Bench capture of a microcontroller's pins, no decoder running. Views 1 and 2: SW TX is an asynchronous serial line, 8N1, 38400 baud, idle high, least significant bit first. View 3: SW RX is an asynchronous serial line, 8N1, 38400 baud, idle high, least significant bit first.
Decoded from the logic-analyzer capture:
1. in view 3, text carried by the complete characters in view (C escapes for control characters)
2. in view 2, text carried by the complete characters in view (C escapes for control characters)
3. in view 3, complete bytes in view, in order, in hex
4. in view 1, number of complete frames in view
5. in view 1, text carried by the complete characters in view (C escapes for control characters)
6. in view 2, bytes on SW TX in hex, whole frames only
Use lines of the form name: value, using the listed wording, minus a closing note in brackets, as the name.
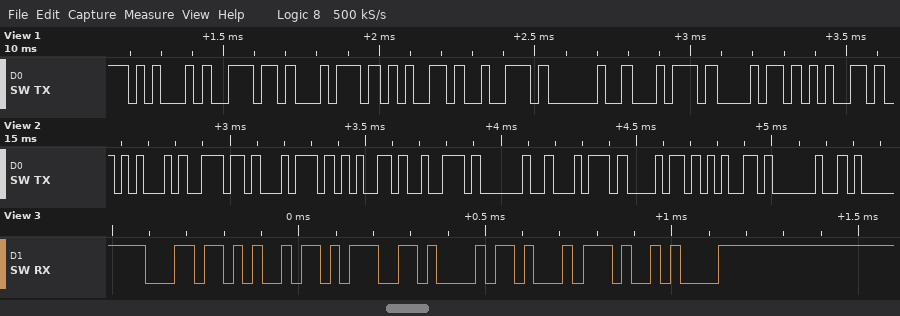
in view 3, text carried by the complete characters in view: "light\n"
in view 2, text carried by the complete characters in view: "Enter the "
in view 3, complete bytes in view, in order, in hex: 6C 69 67 68 74 0A
in view 1, number of complete frames in view: 9
in view 1, text carried by the complete characters in view: "Enter the"
in view 2, bytes on SW TX in hex, whole frames only: 0x45 0x6E 0x74 0x65 0x72 0x20 0x74 0x68 0x65 0x20
